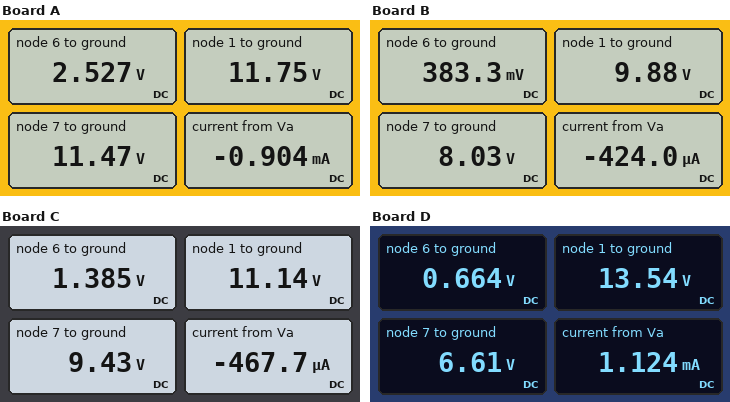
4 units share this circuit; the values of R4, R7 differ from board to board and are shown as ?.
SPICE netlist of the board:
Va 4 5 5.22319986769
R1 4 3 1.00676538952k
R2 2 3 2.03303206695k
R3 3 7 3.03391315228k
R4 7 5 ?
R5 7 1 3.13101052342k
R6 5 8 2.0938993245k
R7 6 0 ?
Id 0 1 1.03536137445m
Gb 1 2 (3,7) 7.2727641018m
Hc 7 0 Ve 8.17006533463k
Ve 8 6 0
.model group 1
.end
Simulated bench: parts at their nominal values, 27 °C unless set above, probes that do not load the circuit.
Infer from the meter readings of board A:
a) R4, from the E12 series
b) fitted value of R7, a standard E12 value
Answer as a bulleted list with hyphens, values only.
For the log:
- 12 kΩ
- 1.8 kΩ
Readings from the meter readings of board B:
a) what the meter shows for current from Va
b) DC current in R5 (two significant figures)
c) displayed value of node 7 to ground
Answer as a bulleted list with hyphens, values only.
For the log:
- -424.0 µA
- 590 µA
- 8.03 V
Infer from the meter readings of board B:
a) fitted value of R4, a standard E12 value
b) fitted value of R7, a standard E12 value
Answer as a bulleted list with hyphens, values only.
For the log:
- 10 kΩ
- 390 Ω
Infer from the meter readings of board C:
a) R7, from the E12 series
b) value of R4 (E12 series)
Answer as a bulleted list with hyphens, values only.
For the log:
- 1.2 kΩ
- 8.2 kΩ
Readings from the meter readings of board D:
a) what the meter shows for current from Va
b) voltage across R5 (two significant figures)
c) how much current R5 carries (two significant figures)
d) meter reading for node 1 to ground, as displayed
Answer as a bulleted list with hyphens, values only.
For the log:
- 1.124 mA
- 6.9 V
- 2.2 mA
- 13.54 V
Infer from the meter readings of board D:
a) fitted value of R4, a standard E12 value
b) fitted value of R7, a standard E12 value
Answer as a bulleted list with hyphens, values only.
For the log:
- 2.2 kΩ
- 820 Ω
